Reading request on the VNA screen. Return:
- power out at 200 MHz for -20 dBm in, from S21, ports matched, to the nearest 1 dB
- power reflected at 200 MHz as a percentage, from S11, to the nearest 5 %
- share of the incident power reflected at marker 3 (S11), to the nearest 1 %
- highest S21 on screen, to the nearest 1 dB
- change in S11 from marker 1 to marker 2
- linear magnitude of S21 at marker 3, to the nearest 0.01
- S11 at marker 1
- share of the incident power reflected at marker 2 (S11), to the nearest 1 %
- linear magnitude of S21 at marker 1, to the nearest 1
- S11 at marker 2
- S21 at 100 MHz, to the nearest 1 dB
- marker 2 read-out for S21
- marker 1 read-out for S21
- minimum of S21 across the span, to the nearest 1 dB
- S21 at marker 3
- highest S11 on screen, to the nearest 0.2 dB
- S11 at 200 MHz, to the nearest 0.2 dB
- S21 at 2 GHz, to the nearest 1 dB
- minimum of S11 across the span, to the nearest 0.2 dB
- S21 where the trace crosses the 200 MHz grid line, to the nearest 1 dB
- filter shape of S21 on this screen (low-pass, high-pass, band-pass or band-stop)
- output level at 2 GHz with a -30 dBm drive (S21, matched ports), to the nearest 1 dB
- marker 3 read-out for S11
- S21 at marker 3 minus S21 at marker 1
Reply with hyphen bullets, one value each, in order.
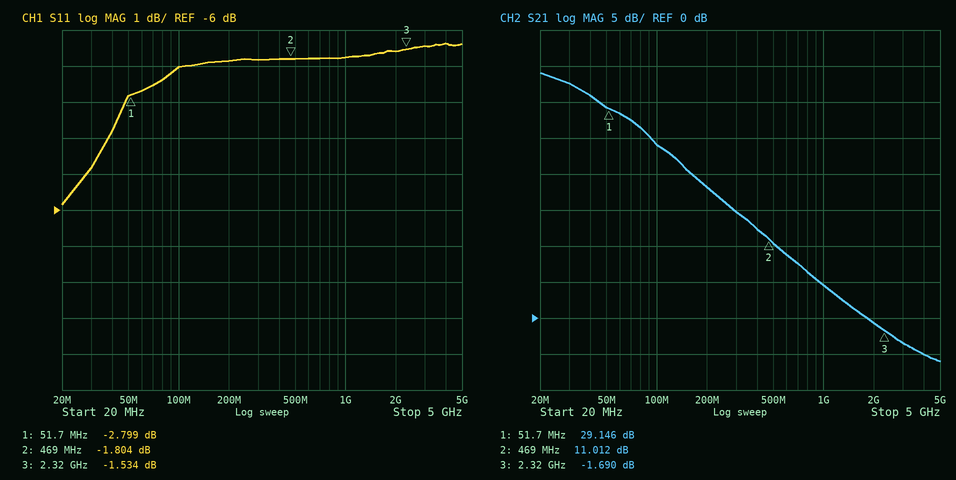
- -2 dBm
- 65 %
- 70 %
- 34 dB
- 0.995 dB
- 0.82
- -2.799 dB
- 66 %
- 29
- -1.804 dB
- 24 dB
- 11.012 dB
- 29.146 dB
- -6 dB
- -1.690 dB
- -1.4 dB
- -1.8 dB
- -1 dB
- -5.8 dB
- 18 dB
- low-pass
- -31 dBm
- -1.534 dB
- -30.836 dB
